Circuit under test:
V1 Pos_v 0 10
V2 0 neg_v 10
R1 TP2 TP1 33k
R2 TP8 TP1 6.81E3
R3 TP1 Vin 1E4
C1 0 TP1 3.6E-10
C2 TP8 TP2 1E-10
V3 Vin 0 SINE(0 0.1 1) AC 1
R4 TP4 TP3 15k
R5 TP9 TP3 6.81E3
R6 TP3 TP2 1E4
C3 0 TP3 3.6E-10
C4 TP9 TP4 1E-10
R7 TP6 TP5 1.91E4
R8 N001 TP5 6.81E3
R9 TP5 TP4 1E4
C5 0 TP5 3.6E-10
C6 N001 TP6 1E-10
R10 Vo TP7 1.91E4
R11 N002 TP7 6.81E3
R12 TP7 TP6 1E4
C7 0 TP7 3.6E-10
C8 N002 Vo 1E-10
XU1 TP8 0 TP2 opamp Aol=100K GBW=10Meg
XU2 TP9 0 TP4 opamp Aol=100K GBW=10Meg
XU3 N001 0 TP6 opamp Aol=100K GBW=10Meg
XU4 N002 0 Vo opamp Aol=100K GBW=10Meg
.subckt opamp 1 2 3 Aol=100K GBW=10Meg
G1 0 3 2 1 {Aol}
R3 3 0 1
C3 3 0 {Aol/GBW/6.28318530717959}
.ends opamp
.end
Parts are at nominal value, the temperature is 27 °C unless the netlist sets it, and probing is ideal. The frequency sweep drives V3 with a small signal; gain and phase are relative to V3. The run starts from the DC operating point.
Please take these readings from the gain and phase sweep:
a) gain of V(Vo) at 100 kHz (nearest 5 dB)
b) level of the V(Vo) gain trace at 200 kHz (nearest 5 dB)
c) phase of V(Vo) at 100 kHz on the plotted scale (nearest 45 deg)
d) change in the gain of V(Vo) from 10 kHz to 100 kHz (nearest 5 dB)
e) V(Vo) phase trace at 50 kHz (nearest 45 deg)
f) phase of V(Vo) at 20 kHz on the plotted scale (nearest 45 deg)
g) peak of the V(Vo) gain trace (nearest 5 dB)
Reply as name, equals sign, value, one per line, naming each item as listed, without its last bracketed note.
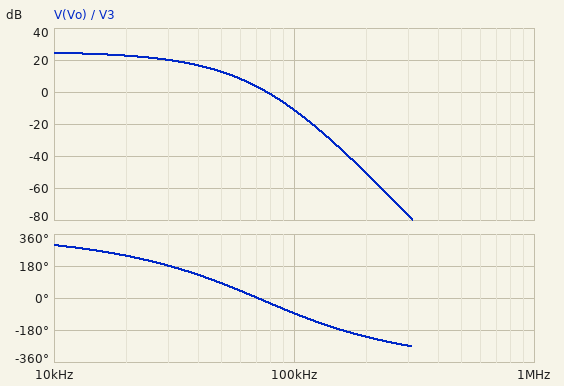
gain of V(Vo) at 100 kHz = -10 dB
level of the V(Vo) gain trace at 200 kHz = -50 dB
phase of V(Vo) at 100 kHz on the plotted scale = -90 deg
change in the gain of V(Vo) from 10 kHz to 100 kHz = -35 dB
V(Vo) phase trace at 50 kHz = 90 deg
phase of V(Vo) at 20 kHz on the plotted scale = 225 deg
peak of the V(Vo) gain trace = 25 dB
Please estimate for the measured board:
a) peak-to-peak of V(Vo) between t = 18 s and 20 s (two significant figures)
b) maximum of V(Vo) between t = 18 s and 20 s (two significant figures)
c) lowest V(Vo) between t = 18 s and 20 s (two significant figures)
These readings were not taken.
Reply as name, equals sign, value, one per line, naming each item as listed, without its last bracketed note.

peak-to-peak of V(Vo) between t = 18 s and 20 s = 3.6 V
maximum of V(Vo) between t = 18 s and 20 s = 1.8 V
lowest V(Vo) between t = 18 s and 20 s = -1.8 V
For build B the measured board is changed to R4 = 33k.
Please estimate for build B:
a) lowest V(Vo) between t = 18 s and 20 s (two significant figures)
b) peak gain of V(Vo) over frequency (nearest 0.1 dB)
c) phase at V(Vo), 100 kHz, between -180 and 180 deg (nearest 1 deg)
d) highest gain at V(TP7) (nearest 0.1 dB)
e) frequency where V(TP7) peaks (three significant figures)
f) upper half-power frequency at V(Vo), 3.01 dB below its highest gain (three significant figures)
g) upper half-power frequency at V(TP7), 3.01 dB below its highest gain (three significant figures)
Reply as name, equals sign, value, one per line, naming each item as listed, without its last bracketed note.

lowest V(Vo) between t = 18 s and 20 s = -4.0 V
peak gain of V(Vo) over frequency = 32.0 dB
phase at V(Vo), 100 kHz, between -180 and 180 deg = -102 deg
highest gain at V(TP7) = 7.4 dB
frequency where V(TP7) peaks = 23.5 kHz
upper half-power frequency at V(Vo), 3.01 dB below its highest gain = 18.2 kHz
upper half-power frequency at V(TP7), 3.01 dB below its highest gain = 41.8 kHz
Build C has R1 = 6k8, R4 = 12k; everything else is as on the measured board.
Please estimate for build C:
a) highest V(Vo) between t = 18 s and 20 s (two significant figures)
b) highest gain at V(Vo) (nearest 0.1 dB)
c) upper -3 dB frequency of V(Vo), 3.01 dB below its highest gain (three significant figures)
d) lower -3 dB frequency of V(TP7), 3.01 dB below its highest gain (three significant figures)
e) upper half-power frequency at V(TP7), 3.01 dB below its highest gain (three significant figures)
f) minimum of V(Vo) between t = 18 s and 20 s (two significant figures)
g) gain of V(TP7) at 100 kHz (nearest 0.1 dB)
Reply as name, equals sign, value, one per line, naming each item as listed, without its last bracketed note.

highest V(Vo) between t = 18 s and 20 s = 300 mV
highest gain at V(Vo) = 9.5 dB
upper -3 dB frequency of V(Vo), 3.01 dB below its highest gain = 35.7 kHz
lower -3 dB frequency of V(TP7), 3.01 dB below its highest gain = 20.4 kHz
upper half-power frequency at V(TP7), 3.01 dB below its highest gain = 68.6 kHz
minimum of V(Vo) between t = 18 s and 20 s = -300 mV
gain of V(TP7) at 100 kHz = -20.7 dB
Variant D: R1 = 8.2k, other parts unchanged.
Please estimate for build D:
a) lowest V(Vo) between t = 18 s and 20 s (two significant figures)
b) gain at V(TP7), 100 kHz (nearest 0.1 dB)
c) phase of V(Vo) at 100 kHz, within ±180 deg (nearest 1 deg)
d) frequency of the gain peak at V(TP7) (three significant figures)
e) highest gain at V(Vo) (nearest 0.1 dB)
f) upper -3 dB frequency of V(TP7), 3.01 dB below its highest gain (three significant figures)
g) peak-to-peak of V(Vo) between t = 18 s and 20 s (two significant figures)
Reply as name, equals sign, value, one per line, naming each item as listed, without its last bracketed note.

lowest V(Vo) between t = 18 s and 20 s = -450 mV
gain at V(TP7), 100 kHz = -19.6 dB
phase of V(Vo) at 100 kHz, within ±180 deg = -47 deg
frequency of the gain peak at V(TP7) = 39.3 kHz
highest gain at V(Vo) = 13.0 dB
upper -3 dB frequency of V(TP7), 3.01 dB below its highest gain = 64.5 kHz
peak-to-peak of V(Vo) between t = 18 s and 20 s = 900 mV
